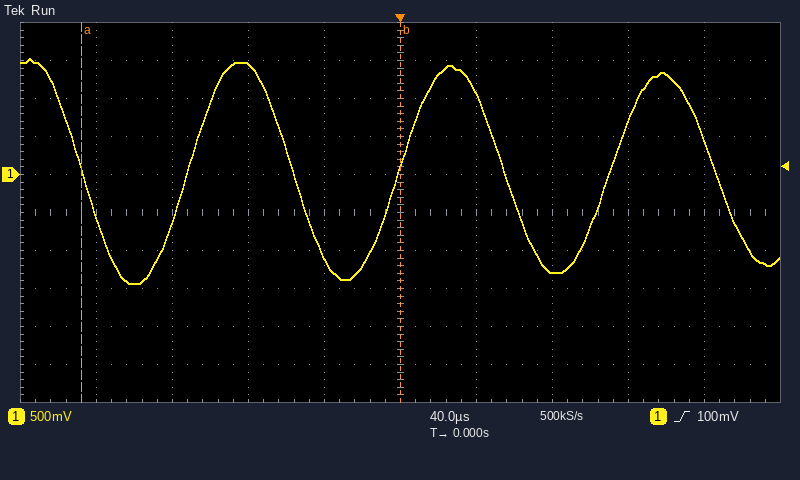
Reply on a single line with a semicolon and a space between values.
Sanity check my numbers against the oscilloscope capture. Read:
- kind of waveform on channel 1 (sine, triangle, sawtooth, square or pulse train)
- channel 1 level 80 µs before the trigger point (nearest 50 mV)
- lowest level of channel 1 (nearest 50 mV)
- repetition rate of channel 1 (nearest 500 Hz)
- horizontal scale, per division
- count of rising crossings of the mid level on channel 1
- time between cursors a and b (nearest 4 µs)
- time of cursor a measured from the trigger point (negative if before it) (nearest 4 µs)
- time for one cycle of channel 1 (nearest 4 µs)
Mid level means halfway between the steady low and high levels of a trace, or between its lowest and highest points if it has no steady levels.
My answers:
sine; 1.45 V; -1.45 V; 9.0 kHz; 40 µs; 3; 168 µs; -168 µs; 112 µs
